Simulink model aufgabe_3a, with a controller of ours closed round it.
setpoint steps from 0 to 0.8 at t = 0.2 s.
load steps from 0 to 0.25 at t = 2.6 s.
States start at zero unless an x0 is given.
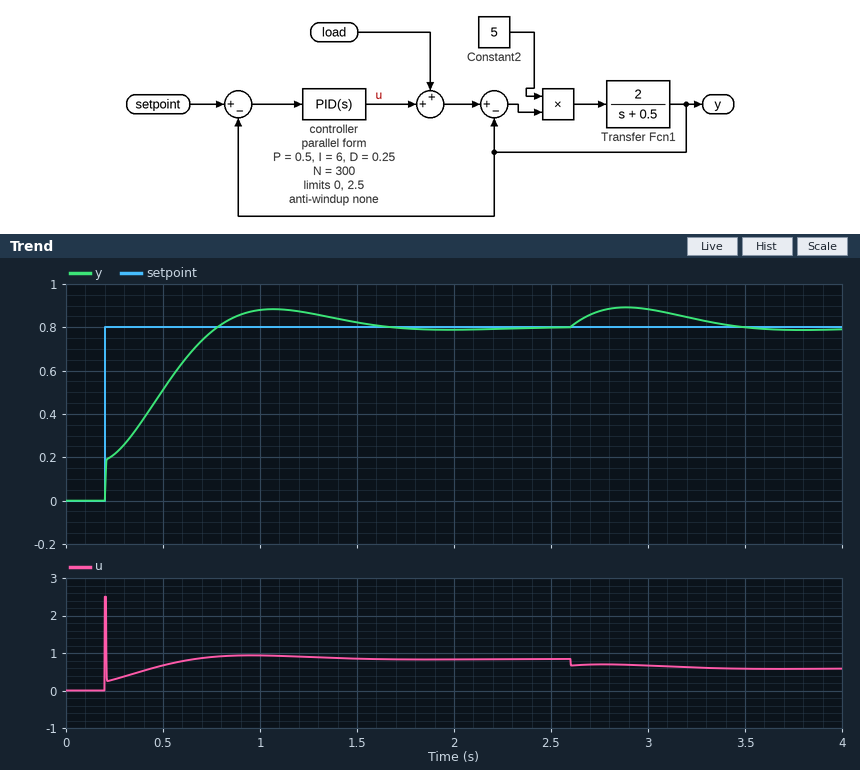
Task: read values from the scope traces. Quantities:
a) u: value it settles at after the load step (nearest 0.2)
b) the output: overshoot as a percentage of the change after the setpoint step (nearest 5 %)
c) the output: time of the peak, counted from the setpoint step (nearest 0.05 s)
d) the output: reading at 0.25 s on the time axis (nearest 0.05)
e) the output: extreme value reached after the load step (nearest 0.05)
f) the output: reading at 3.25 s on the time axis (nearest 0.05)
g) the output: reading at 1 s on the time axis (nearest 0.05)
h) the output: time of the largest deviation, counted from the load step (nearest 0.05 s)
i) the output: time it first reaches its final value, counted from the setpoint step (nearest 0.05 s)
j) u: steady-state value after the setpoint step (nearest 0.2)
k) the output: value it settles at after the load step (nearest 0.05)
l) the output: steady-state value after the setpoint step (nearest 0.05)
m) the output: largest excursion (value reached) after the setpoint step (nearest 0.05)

0.6
10 %
0.85 s
0.20
0.90
0.85
0.90
0.30 s
0.60 s
0.8
0.80
0.80
0.90
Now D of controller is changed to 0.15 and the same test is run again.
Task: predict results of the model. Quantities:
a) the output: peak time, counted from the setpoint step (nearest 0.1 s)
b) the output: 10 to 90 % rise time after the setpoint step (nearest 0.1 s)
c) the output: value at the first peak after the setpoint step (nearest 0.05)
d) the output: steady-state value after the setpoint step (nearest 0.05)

0.8 s
0.4 s
0.85
0.80
